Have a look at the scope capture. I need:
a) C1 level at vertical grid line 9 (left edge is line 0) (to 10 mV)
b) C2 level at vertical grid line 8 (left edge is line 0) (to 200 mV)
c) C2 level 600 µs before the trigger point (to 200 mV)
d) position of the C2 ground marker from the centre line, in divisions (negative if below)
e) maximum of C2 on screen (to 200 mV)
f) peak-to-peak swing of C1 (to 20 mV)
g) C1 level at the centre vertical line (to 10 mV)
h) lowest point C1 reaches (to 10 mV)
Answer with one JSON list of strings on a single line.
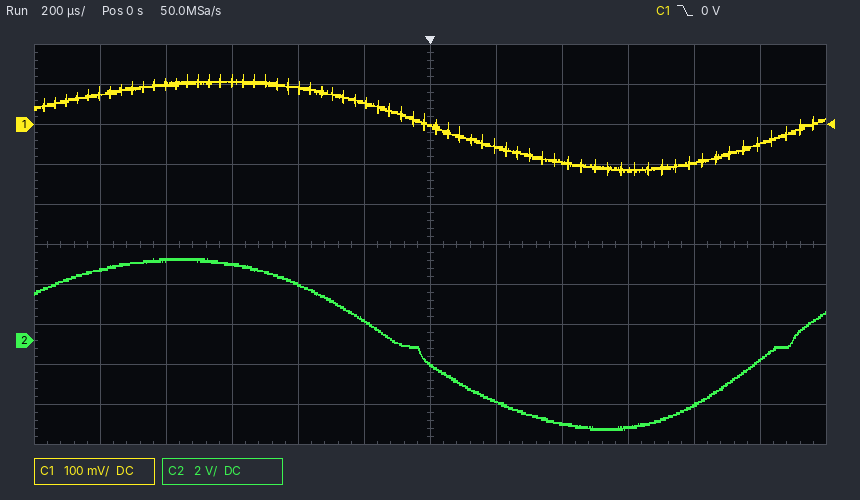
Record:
["-110 mV", "-4.2 V", "3.8 V", "-2.4 div", "4.0 V", "260 mV", "-10 mV", "-130 mV"]
